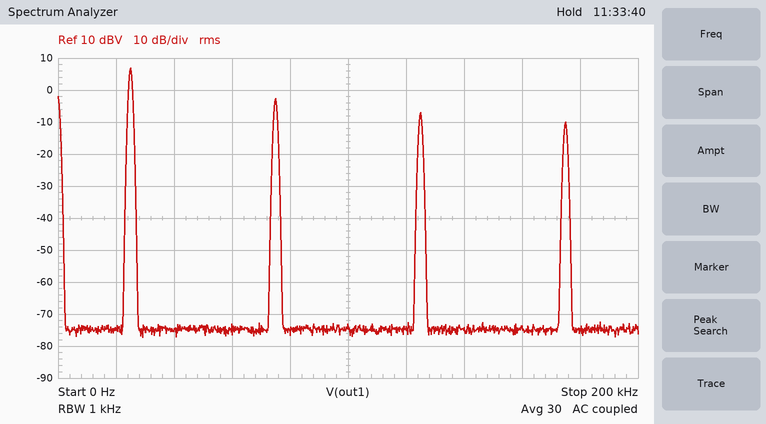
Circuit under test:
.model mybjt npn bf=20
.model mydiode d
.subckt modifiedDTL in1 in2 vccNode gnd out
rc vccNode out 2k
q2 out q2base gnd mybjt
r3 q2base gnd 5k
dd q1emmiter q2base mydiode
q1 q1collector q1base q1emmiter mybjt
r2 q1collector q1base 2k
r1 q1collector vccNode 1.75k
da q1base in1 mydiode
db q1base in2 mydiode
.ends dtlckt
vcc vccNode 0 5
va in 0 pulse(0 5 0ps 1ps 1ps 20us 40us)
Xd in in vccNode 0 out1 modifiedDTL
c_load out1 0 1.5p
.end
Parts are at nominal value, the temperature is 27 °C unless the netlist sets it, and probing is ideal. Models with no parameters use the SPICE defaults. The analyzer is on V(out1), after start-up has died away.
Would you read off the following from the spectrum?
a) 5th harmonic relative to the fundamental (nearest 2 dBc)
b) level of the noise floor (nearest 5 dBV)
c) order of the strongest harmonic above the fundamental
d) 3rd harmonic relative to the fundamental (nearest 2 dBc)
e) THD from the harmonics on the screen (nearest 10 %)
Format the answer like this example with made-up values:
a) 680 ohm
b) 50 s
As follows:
a) -14 dBc
b) -75 dBV
c) 3
d) -10 dBc
e) 40 %
